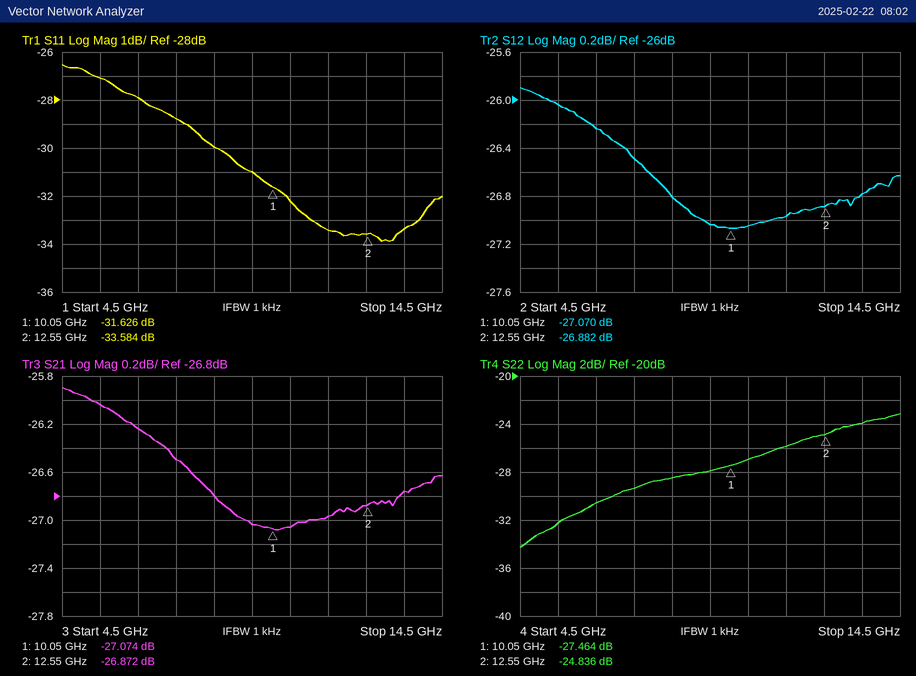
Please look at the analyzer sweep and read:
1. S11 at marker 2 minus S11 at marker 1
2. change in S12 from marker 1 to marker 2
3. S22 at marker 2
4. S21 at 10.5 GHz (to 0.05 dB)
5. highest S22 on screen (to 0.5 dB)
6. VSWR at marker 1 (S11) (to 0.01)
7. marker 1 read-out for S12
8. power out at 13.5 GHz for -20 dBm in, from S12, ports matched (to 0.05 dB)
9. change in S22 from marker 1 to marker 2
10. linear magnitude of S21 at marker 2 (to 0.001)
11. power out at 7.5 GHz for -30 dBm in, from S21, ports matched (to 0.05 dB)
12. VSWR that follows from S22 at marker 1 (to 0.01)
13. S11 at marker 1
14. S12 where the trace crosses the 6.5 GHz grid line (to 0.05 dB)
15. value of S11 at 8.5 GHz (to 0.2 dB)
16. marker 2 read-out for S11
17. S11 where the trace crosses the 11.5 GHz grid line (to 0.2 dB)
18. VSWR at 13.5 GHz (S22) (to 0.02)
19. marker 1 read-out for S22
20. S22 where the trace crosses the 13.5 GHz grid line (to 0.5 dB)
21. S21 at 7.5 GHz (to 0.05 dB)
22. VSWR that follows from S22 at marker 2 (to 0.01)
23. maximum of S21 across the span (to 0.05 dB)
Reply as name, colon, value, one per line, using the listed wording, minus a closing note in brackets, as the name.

S11 at marker 2 minus S11 at marker 1: -1.958 dB
change in S12 from marker 1 to marker 2: 0.188 dB
S22 at marker 2: -24.836 dB
S21 at 10.5 GHz: -27.05 dB
highest S22 on screen: -23.0 dB
VSWR at marker 1 (S11): 1.05
marker 1 read-out for S12: -27.070 dB
power out at 13.5 GHz for -20 dBm in, from S12, ports matched: -46.80 dBm
change in S22 from marker 1 to marker 2: 2.628 dB
linear magnitude of S21 at marker 2: 0.045
power out at 7.5 GHz for -30 dBm in, from S21, ports matched: -56.50 dBm
VSWR that follows from S22 at marker 1: 1.09
S11 at marker 1: -31.626 dB
S12 where the trace crosses the 6.5 GHz grid line: -26.25 dB
value of S11 at 8.5 GHz: -30.0 dB
marker 2 read-out for S11: -33.584 dB
S11 where the trace crosses the 11.5 GHz grid line: -33.4 dB
VSWR at 13.5 GHz (S22): 1.14
marker 1 read-out for S22: -27.464 dB
S22 where the trace crosses the 13.5 GHz grid line: -24.0 dB
S21 at 7.5 GHz: -26.50 dB
VSWR that follows from S22 at marker 2: 1.12
maximum of S21 across the span: -25.90 dB
